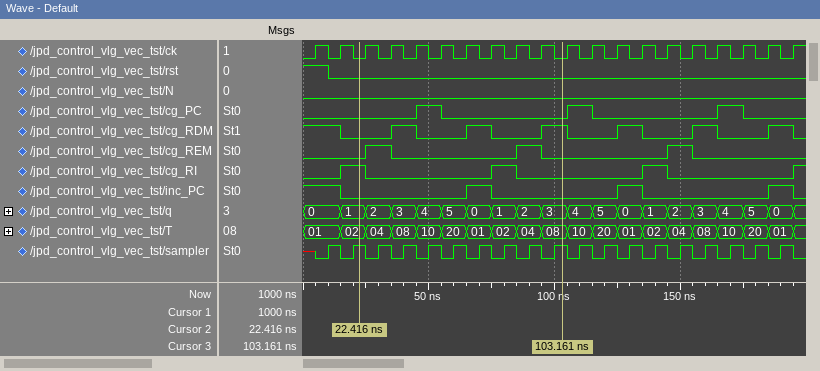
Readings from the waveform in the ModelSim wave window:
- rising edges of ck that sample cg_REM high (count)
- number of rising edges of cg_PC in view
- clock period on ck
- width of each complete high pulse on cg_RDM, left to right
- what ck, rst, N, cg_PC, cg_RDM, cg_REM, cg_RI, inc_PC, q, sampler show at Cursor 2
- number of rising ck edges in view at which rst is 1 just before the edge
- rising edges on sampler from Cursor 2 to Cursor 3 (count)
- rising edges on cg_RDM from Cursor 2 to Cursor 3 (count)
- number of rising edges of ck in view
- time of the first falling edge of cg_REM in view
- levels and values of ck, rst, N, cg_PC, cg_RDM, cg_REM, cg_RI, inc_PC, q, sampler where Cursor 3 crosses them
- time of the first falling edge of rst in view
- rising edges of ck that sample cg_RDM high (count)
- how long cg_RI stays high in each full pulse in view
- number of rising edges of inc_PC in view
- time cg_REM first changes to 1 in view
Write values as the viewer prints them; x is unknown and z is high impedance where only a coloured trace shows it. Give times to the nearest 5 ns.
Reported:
3
3
10 ns
10 ns, 10 ns, 10 ns, 10 ns, 10 ns, 10 ns
ck=0, rst=0, N=0, cg_PC=0, cg_RDM=0, cg_REM=0, cg_RI=1, inc_PC=0, q=1, sampler=1
1
8
3
20
35 ns
ck=0, rst=0, N=0, cg_PC=0, cg_RDM=1, cg_REM=0, cg_RI=0, inc_PC=0, q=3, sampler=1
10 ns
8
10 ns, 10 ns, 10 ns
3
25 ns
